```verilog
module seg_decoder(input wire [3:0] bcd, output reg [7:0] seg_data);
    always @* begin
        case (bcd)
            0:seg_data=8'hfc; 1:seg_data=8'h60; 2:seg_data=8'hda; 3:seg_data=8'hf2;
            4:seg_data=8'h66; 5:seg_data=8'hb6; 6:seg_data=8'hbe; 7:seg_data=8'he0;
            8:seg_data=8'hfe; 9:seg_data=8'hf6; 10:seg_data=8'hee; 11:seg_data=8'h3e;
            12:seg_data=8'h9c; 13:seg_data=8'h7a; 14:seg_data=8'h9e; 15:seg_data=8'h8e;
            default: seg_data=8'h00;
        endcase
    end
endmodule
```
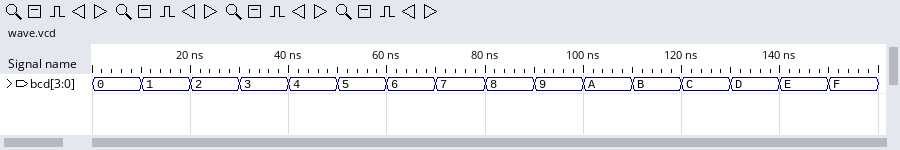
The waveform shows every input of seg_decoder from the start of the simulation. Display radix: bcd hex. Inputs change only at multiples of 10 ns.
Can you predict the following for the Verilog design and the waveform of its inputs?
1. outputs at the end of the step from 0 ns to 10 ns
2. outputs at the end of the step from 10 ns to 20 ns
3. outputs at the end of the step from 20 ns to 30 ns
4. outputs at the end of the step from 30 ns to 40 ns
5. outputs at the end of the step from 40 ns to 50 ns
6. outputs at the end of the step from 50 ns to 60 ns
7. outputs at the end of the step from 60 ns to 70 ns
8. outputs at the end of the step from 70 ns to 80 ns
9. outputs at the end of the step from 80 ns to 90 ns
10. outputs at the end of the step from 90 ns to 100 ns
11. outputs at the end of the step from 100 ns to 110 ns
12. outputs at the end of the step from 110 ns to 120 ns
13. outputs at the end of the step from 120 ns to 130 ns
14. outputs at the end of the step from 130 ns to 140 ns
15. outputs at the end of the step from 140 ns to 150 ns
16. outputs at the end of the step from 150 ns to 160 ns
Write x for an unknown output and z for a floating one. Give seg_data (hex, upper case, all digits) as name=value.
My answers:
seg_data=FC
seg_data=60
seg_data=DA
seg_data=F2
seg_data=66
seg_data=B6
seg_data=BE
seg_data=E0
seg_data=FE
seg_data=F6
seg_data=EE
seg_data=3E
seg_data=9C
seg_data=7A
seg_data=9E
seg_data=8E
